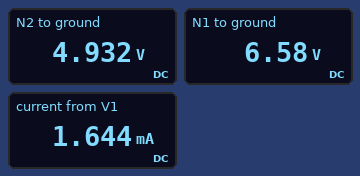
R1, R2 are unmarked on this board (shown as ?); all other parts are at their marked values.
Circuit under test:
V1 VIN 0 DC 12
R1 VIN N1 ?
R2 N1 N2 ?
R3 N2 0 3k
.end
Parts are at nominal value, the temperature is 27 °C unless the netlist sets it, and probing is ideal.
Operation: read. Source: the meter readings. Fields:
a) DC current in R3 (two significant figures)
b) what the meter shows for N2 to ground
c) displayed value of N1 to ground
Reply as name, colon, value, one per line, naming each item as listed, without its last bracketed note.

DC current in R3: 1.6 mA
what the meter shows for N2 to ground: 4.932 V
displayed value of N1 to ground: 6.58 V
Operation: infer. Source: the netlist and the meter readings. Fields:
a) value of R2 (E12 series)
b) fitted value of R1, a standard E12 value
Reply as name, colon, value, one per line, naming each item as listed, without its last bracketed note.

value of R2: 1 kΩ
fitted value of R1, a standard E12 value: 3.3 kΩ
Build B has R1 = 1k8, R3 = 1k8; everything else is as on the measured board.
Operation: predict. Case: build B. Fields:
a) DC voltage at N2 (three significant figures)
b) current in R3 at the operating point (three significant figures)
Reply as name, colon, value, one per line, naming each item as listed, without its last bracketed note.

DC voltage at N2: 4.70 V
current in R3 at the operating point: 2.61 mA
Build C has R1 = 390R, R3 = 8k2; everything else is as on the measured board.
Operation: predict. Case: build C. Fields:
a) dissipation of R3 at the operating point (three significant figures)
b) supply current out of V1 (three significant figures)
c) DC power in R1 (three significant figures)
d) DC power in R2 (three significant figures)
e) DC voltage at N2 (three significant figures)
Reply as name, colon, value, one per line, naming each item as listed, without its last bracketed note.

dissipation of R3 at the operating point: 12.8 mW
supply current out of V1: 1.25 mA
DC power in R1: 611 µW
DC power in R2: 1.57 mW
DC voltage at N2: 10.3 V
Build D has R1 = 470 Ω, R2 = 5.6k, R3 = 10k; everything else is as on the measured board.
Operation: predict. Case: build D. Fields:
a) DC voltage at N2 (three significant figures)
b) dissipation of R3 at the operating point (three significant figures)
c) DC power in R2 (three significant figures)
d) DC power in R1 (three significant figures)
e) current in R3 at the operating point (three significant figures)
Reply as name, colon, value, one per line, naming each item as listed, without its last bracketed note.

DC voltage at N2: 7.47 V
dissipation of R3 at the operating point: 5.58 mW
DC power in R2: 3.12 mW
DC power in R1: 262 µW
current in R3 at the operating point: 747 µA
